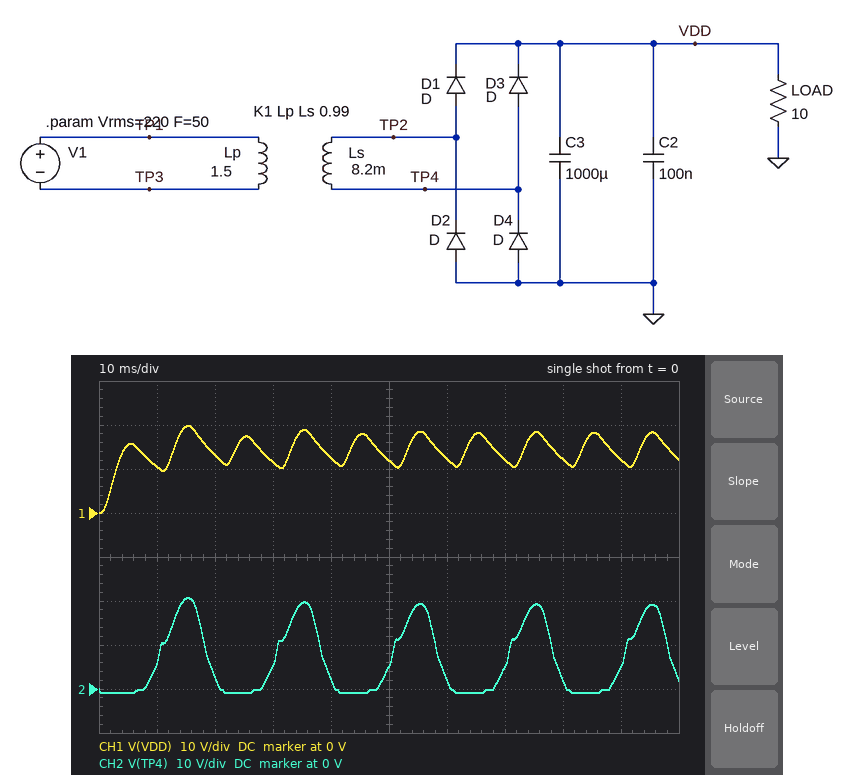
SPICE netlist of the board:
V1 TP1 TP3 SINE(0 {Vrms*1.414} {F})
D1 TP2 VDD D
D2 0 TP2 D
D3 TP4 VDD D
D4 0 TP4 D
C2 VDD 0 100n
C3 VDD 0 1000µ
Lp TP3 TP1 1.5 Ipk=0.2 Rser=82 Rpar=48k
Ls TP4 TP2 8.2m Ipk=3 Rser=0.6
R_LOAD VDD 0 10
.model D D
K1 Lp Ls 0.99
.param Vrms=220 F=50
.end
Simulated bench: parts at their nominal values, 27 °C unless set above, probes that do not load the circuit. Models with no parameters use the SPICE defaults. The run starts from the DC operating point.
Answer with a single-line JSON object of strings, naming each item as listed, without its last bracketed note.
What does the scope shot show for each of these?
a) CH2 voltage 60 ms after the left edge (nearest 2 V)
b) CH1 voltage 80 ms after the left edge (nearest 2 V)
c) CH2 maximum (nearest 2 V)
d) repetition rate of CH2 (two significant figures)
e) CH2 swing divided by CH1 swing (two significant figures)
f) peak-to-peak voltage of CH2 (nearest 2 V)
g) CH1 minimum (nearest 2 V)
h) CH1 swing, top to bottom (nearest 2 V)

{"CH2 voltage 60 ms after the left edge": "2 V", "CH1 voltage 80 ms after the left edge": "12 V", "CH2 maximum": "20 V", "repetition rate of CH2": "50 Hz", "CH2 swing divided by CH1 swing": "1.1", "peak-to-peak voltage of CH2": "22 V", "CH1 minimum": "0 V", "CH1 swing, top to bottom": "20 V"}
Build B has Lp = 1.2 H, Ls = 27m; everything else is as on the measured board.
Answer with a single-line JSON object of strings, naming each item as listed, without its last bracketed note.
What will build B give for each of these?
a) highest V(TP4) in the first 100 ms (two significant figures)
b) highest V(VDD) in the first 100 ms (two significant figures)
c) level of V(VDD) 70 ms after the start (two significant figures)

{"highest V(TP4) in the first 100 ms": "35 V", "highest V(VDD) in the first 100 ms": "34 V", "level of V(VDD) 70 ms after the start": "23 V"}
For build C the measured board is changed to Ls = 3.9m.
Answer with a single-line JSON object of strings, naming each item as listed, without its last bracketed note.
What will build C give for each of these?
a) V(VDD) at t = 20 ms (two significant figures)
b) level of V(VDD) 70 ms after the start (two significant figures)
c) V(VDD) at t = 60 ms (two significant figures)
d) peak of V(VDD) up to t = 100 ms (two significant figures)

{"V(VDD) at t = 20 ms": "8.8 V", "level of V(VDD) 70 ms after the start": "8.1 V", "V(VDD) at t = 60 ms": "8.2 V", "peak of V(VDD) up to t = 100 ms": "14 V"}
